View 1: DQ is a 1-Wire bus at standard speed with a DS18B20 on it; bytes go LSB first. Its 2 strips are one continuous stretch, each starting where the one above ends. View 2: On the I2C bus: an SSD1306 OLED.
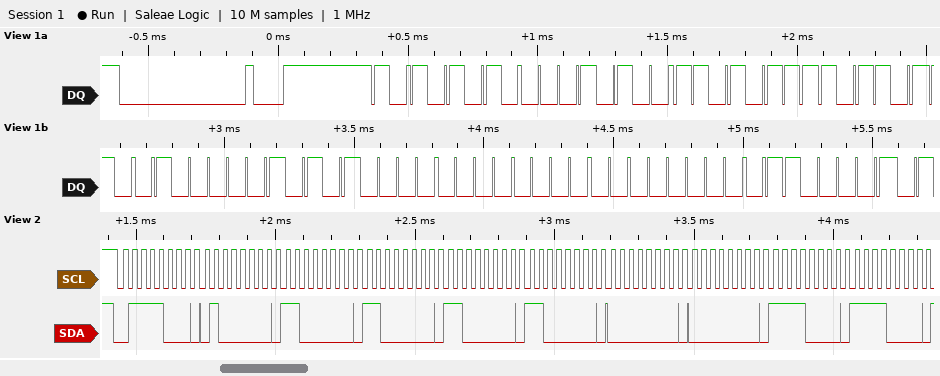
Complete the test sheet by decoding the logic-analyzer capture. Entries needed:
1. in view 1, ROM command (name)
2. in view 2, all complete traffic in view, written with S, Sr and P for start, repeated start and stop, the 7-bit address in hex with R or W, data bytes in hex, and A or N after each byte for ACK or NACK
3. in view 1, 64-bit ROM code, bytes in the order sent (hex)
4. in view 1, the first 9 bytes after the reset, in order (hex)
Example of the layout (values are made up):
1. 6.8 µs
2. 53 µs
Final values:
1. Match ROM
2. S 3CW A 40 A C0 A C0 A C0 A C0 A 00 A 00 A F0 A F0 A
3. 28 EB 6D 82 0A 00 00 86
4. 55 28 EB 6D 82 0A 00 00 86
